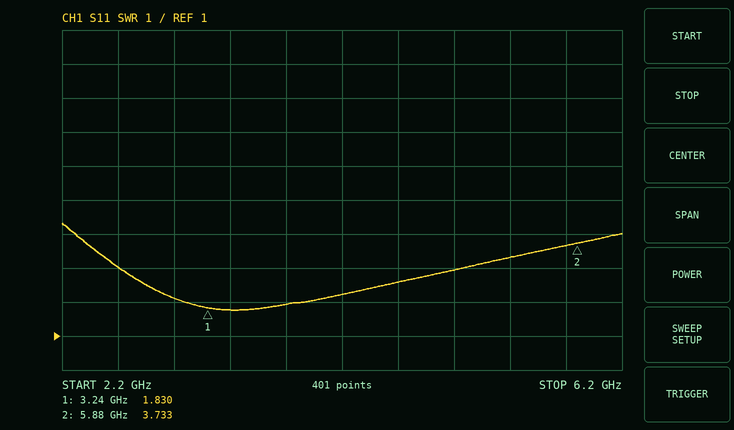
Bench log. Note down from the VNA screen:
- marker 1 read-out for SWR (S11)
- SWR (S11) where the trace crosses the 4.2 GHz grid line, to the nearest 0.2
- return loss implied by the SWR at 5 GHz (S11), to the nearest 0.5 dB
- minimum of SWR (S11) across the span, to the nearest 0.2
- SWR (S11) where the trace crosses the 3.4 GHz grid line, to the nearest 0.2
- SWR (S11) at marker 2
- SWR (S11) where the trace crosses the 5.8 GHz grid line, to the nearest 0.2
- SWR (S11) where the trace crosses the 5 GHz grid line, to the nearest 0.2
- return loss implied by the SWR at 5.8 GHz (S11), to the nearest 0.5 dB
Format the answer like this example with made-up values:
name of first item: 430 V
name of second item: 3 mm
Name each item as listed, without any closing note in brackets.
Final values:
marker 1 read-out for SWR: 1.830
SWR (S11) where the trace crosses the 4.2 GHz grid line, to the nearest 0.2: 2.2
return loss implied by the SWR at 5 GHz (S11), to the nearest 0.5 dB: 6.0 dB
minimum of SWR (S11) across the span, to the nearest 0.2: 1.8
SWR (S11) where the trace crosses the 3.4 GHz grid line, to the nearest 0.2: 1.8
SWR (S11) at marker 2: 3.733
SWR (S11) where the trace crosses the 5.8 GHz grid line, to the nearest 0.2: 3.6
SWR (S11) where the trace crosses the 5 GHz grid line, to the nearest 0.2: 3.0
return loss implied by the SWR at 5.8 GHz (S11), to the nearest 0.5 dB: 5.0 dB
